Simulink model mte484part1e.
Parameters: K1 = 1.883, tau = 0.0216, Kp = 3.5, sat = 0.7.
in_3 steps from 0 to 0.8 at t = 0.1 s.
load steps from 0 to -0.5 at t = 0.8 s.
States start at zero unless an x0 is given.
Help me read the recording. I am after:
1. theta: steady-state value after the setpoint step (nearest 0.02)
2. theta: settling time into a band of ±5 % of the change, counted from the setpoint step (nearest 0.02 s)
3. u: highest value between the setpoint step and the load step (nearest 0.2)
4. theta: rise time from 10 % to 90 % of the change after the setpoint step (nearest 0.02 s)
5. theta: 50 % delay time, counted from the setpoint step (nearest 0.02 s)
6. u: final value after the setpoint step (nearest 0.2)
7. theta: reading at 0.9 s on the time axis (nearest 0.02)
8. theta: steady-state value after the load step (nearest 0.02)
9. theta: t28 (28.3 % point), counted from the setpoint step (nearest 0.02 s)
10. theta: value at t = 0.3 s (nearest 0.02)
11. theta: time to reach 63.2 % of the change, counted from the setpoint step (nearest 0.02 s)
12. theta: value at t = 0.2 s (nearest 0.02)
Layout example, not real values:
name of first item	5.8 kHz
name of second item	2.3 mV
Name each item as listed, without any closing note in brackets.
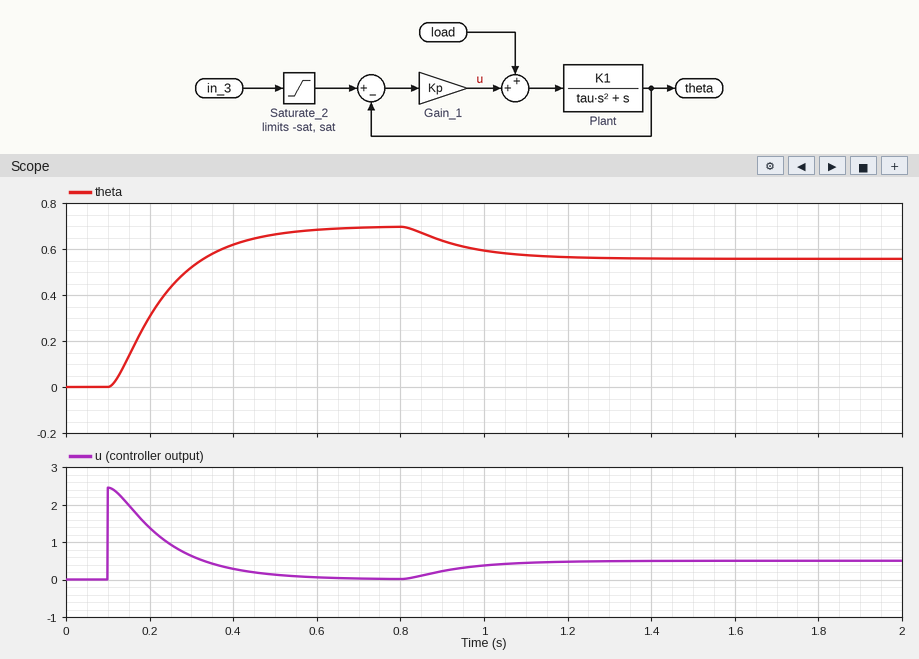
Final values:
theta: steady-state value after the setpoint step	0.70
theta: settling time into a band of ±5 % of the change, counted from the setpoint step	0.40 s
u: highest value between the setpoint step and the load step	2.4
theta: rise time from 10 % to 90 % of the change after the setpoint step	0.28 s
theta: 50 % delay time, counted from the setpoint step	0.12 s
u: final value after the setpoint step	0.0
theta: reading at 0.9 s on the time axis	0.64
theta: steady-state value after the load step	0.56
theta: t28 (28.3 % point), counted from the setpoint step	0.06 s
theta: value at t = 0.3 s	0.52
theta: time to reach 63.2 % of the change, counted from the setpoint step	0.16 s
theta: value at t = 0.2 s	0.30
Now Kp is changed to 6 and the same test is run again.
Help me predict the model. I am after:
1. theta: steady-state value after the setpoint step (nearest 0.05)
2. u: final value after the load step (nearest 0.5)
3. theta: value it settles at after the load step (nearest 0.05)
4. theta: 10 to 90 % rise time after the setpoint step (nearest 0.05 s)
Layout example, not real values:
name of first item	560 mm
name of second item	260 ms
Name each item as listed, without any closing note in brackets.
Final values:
theta: steady-state value after the setpoint step	0.70
u: final value after the load step	0.5
theta: value it settles at after the load step	0.60
theta: 10 to 90 % rise time after the setpoint step	0.15 s
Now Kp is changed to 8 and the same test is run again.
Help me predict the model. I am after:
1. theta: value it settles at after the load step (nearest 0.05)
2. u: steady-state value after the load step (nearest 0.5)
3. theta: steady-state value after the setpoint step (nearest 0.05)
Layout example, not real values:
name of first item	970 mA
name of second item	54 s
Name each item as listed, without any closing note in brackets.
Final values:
theta: value it settles at after the load step	0.65
u: steady-state value after the load step	0.5
theta: steady-state value after the setpoint step	0.70
